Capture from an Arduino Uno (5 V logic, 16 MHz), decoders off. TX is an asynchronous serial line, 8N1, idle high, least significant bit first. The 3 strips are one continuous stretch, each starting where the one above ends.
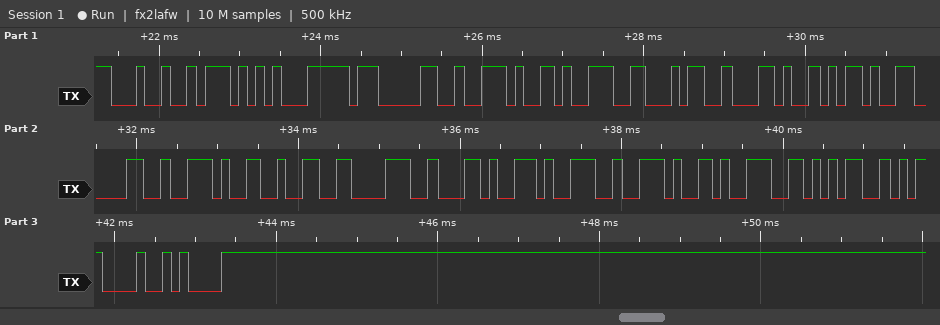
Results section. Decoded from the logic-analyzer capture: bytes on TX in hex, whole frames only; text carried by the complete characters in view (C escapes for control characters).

24 57 7C 30 2E 39 34 2C 2D 30 2E 32 38 2C 39 2E 39 35 0D 0A
"$W|0.94,-0.28,9.95\r\n"
